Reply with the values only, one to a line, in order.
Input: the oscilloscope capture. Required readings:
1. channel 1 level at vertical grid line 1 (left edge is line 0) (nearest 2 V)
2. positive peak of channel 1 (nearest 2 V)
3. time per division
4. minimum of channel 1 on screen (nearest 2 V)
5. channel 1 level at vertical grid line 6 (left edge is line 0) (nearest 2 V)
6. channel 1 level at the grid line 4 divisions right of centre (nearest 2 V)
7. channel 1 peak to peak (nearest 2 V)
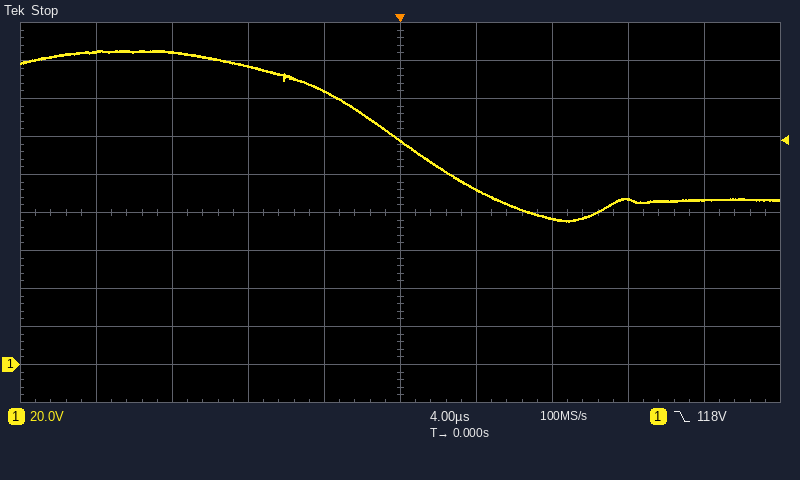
164 V
166 V
4 µs
76 V
92 V
86 V
90 V
